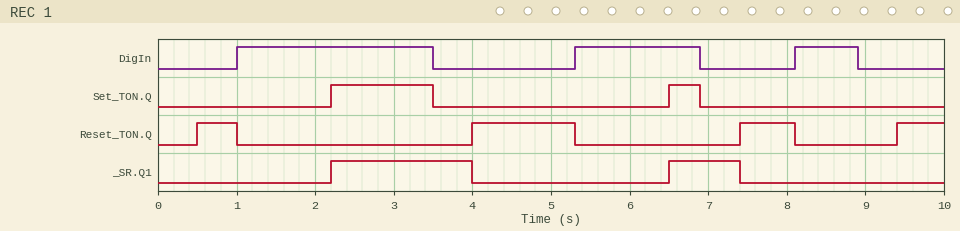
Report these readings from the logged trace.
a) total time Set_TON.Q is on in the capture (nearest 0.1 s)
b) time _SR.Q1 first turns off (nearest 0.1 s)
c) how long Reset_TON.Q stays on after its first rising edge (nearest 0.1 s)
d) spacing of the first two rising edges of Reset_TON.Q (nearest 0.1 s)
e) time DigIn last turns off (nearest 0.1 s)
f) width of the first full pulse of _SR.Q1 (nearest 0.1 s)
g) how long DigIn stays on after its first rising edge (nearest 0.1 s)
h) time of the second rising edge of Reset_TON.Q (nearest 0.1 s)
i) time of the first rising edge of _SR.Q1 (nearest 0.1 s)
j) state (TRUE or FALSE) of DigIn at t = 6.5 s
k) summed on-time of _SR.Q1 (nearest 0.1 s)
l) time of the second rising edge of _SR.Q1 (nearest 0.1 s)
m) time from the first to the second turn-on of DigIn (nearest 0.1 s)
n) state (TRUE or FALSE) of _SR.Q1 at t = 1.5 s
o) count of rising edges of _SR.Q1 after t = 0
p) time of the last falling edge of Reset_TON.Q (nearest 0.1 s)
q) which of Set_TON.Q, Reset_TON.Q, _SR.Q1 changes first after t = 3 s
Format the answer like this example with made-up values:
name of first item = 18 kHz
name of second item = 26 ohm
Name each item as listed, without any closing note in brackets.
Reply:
total time Set_TON.Q is on in the capture = 1.7 s
time _SR.Q1 first turns off = 4.0 s
how long Reset_TON.Q stays on after its first rising edge = 0.5 s
spacing of the first two rising edges of Reset_TON.Q = 3.5 s
time DigIn last turns off = 8.9 s
width of the first full pulse of _SR.Q1 = 1.8 s
how long DigIn stays on after its first rising edge = 2.5 s
time of the second rising edge of Reset_TON.Q = 4.0 s
time of the first rising edge of _SR.Q1 = 2.2 s
state (TRUE or FALSE) of DigIn at t = 6.5 s = TRUE
summed on-time of _SR.Q1 = 2.7 s
time of the second rising edge of _SR.Q1 = 6.5 s
time from the first to the second turn-on of DigIn = 4.3 s
state (TRUE or FALSE) of _SR.Q1 at t = 1.5 s = FALSE
count of rising edges of _SR.Q1 after t = 0 = 2
time of the last falling edge of Reset_TON.Q = 8.1 s
which of Set_TON.Q, Reset_TON.Q, _SR.Q1 changes first after t = 3 s = Set_TON.Q
